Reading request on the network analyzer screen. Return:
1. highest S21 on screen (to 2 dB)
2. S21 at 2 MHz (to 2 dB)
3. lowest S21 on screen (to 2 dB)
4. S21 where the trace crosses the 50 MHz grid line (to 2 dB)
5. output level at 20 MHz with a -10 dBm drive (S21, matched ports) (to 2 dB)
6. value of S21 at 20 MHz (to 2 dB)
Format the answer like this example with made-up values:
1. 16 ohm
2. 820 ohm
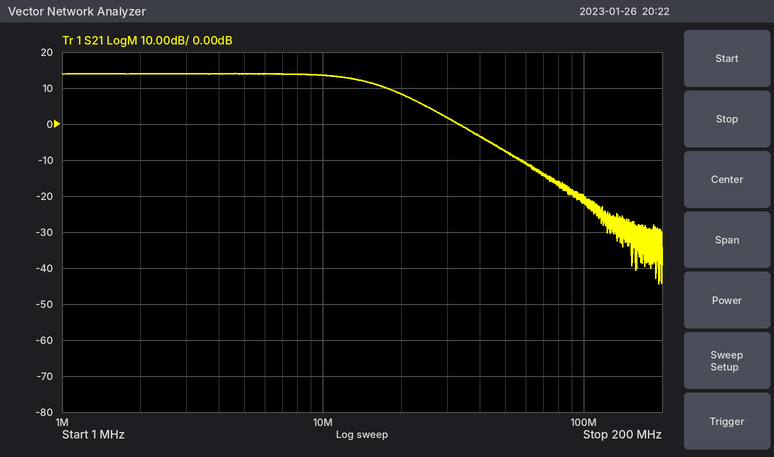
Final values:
1. 14 dB
2. 14 dB
3. -44 dB
4. -8 dB
5. -2 dBm
6. 8 dB
